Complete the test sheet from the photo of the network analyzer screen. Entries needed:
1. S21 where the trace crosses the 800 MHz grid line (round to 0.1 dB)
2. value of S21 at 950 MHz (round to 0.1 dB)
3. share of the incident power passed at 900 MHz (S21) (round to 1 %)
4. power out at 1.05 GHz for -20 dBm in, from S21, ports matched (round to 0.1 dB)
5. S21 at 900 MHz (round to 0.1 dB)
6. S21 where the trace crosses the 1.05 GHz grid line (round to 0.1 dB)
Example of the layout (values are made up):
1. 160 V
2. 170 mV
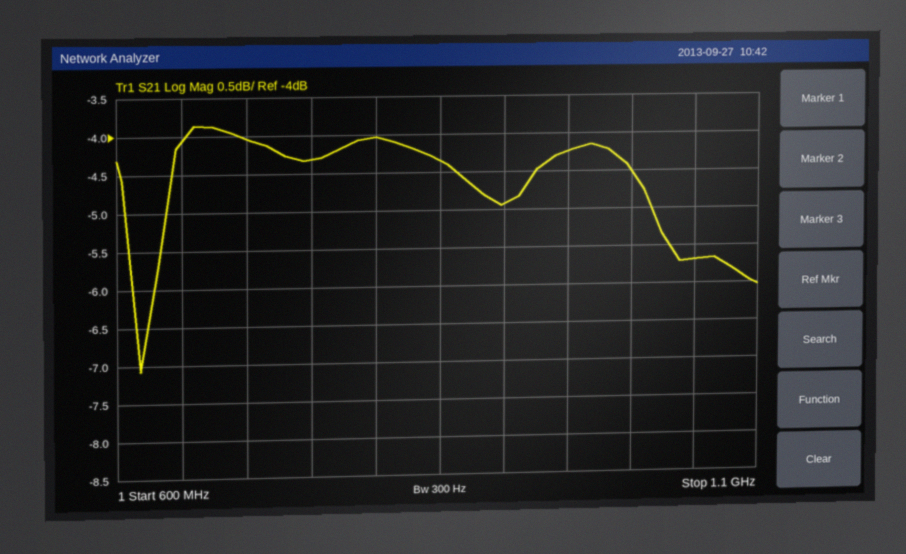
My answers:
1. -4.0 dB
2. -4.2 dB
3. 32 %
4. -25.7 dBm
5. -4.9 dB
6. -5.7 dB
